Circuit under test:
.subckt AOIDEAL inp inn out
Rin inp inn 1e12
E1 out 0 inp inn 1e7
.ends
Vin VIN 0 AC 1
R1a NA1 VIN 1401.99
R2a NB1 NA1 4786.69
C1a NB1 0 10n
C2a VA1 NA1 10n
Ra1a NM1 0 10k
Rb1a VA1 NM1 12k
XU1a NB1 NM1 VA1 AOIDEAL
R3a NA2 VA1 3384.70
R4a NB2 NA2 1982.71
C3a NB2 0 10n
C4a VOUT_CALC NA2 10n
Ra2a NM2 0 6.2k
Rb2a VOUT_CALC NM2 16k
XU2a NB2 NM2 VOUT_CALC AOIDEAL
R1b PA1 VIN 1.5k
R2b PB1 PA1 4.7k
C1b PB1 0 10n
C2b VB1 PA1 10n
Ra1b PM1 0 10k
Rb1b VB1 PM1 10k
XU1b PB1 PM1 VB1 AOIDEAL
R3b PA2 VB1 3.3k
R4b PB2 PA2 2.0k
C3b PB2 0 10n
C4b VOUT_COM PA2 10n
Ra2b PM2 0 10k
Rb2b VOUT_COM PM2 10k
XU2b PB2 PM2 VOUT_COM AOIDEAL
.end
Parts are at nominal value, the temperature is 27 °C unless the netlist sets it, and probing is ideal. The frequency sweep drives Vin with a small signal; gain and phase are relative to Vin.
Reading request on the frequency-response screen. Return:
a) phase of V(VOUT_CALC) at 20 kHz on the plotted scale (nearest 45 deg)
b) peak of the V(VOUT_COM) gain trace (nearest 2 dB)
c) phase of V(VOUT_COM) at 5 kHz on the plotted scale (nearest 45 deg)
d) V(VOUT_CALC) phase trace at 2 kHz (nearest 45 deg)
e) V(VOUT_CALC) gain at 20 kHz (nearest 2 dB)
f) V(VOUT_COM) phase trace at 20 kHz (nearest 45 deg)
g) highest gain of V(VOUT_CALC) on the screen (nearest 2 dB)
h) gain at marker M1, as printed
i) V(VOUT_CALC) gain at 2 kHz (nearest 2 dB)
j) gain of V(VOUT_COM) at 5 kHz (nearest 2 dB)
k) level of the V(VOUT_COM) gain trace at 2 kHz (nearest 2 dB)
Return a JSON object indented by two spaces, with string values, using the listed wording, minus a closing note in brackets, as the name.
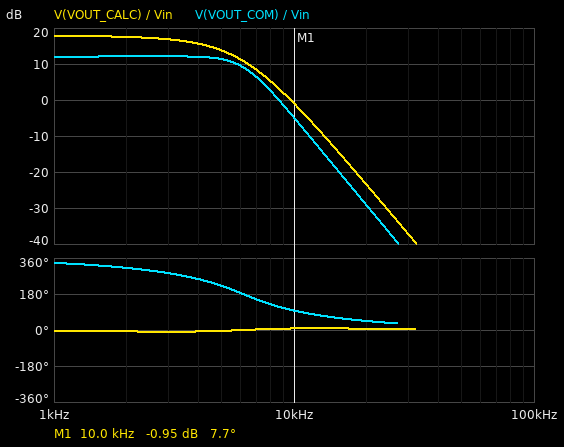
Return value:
{
  "phase of V(VOUT_CALC) at 20 kHz on the plotted scale": "0 deg",
  "peak of the V(VOUT_COM) gain trace": "12 dB",
  "phase of V(VOUT_COM) at 5 kHz on the plotted scale": "225 deg",
  "V(VOUT_CALC) phase trace at 2 kHz": "0 deg",
  "V(VOUT_CALC) gain at 20 kHz": "-24 dB",
  "V(VOUT_COM) phase trace at 20 kHz": "45 deg",
  "highest gain of V(VOUT_CALC) on the screen": "18 dB",
  "gain at marker M1, as printed": "-0.95 dB",
  "V(VOUT_CALC) gain at 2 kHz": "18 dB",
  "gain of V(VOUT_COM) at 5 kHz": "12 dB",
  "level of the V(VOUT_COM) gain trace at 2 kHz": "12 dB"
}
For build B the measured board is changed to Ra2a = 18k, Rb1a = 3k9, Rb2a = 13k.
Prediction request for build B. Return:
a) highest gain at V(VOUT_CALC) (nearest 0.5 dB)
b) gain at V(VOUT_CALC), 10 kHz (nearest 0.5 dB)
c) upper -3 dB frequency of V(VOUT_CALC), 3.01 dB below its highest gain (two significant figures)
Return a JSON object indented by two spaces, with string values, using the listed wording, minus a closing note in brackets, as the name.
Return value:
{
  "highest gain at V(VOUT_CALC)": "7.5 dB",
  "gain at V(VOUT_CALC), 10 kHz": "-12.0 dB",
  "upper -3 dB frequency of V(VOUT_CALC), 3.01 dB below its highest gain": "3.9 kHz"
}
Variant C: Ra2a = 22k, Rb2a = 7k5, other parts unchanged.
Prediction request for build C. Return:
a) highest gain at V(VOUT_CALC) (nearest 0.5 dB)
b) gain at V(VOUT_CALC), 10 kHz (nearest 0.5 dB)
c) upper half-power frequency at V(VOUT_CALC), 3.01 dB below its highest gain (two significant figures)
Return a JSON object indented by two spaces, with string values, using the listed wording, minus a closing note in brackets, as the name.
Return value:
{
  "highest gain at V(VOUT_CALC)": "9.5 dB",
  "gain at V(VOUT_CALC), 10 kHz": "-11.0 dB",
  "upper half-power frequency at V(VOUT_CALC), 3.01 dB below its highest gain": "3.6 kHz"
}
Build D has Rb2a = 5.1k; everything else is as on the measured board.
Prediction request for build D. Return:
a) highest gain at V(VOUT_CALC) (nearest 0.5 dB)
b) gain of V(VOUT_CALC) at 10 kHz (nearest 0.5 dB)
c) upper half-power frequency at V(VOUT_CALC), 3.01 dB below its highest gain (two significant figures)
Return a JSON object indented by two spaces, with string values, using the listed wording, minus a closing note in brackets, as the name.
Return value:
{
  "highest gain at V(VOUT_CALC)": "12.0 dB",
  "gain of V(VOUT_CALC) at 10 kHz": "-5.5 dB",
  "upper half-power frequency at V(VOUT_CALC), 3.01 dB below its highest gain": "5.4 kHz"
}
